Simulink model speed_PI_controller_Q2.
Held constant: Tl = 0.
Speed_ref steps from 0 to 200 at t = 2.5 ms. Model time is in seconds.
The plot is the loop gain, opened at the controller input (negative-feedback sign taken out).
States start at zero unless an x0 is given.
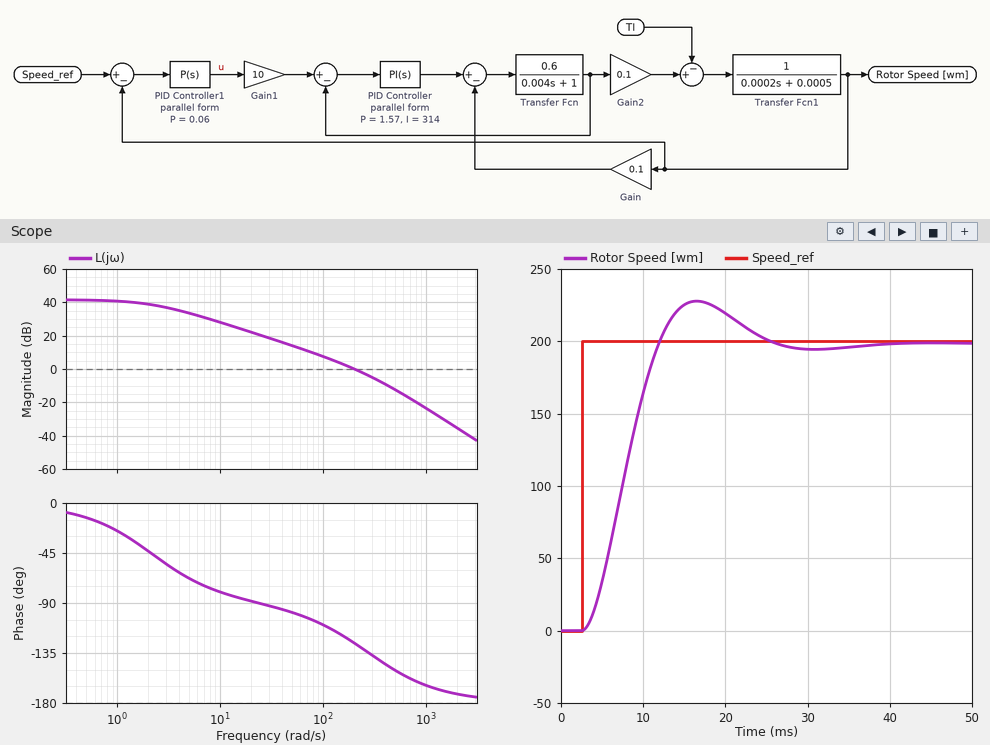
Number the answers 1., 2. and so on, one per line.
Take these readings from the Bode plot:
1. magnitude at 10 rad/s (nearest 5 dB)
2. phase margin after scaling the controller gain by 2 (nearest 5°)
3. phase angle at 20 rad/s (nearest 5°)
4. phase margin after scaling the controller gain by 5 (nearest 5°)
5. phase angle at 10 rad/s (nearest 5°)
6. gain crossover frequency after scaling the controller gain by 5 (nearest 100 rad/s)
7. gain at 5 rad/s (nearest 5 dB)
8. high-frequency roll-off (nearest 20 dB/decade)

1. 30 dB
2. 40°
3. -90°
4. 25°
5. -80°
6. 600 rad/s
7. 35 dB
8. -40 dB/decade
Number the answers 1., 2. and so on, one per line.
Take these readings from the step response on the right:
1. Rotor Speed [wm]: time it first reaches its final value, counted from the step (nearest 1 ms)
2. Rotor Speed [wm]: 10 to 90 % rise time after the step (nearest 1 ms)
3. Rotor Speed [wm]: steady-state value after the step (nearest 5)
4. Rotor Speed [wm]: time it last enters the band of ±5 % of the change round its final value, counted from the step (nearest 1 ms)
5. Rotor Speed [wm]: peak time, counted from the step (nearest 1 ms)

1. 9 ms
2. 6 ms
3. 200
4. 20 ms
5. 14 ms
